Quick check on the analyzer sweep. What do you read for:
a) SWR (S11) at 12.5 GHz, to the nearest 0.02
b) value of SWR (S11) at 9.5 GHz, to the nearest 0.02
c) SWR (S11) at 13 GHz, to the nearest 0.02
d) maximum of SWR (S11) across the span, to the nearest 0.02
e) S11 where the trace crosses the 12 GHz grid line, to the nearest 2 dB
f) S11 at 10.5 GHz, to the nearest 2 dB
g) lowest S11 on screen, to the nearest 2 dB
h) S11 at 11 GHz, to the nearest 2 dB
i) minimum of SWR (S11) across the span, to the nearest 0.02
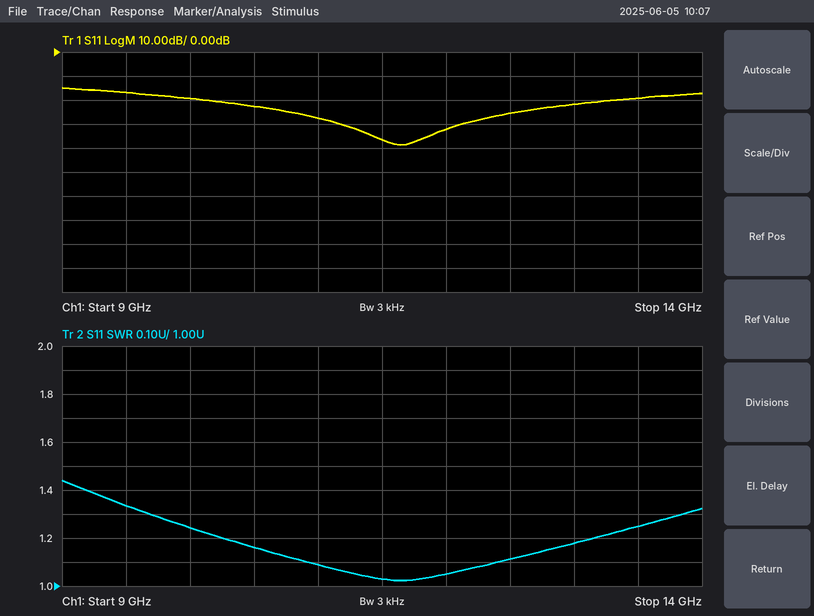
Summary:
1.12
1.34
1.18
1.44
-32 dB
-22 dB
-38 dB
-28 dB
1.02
